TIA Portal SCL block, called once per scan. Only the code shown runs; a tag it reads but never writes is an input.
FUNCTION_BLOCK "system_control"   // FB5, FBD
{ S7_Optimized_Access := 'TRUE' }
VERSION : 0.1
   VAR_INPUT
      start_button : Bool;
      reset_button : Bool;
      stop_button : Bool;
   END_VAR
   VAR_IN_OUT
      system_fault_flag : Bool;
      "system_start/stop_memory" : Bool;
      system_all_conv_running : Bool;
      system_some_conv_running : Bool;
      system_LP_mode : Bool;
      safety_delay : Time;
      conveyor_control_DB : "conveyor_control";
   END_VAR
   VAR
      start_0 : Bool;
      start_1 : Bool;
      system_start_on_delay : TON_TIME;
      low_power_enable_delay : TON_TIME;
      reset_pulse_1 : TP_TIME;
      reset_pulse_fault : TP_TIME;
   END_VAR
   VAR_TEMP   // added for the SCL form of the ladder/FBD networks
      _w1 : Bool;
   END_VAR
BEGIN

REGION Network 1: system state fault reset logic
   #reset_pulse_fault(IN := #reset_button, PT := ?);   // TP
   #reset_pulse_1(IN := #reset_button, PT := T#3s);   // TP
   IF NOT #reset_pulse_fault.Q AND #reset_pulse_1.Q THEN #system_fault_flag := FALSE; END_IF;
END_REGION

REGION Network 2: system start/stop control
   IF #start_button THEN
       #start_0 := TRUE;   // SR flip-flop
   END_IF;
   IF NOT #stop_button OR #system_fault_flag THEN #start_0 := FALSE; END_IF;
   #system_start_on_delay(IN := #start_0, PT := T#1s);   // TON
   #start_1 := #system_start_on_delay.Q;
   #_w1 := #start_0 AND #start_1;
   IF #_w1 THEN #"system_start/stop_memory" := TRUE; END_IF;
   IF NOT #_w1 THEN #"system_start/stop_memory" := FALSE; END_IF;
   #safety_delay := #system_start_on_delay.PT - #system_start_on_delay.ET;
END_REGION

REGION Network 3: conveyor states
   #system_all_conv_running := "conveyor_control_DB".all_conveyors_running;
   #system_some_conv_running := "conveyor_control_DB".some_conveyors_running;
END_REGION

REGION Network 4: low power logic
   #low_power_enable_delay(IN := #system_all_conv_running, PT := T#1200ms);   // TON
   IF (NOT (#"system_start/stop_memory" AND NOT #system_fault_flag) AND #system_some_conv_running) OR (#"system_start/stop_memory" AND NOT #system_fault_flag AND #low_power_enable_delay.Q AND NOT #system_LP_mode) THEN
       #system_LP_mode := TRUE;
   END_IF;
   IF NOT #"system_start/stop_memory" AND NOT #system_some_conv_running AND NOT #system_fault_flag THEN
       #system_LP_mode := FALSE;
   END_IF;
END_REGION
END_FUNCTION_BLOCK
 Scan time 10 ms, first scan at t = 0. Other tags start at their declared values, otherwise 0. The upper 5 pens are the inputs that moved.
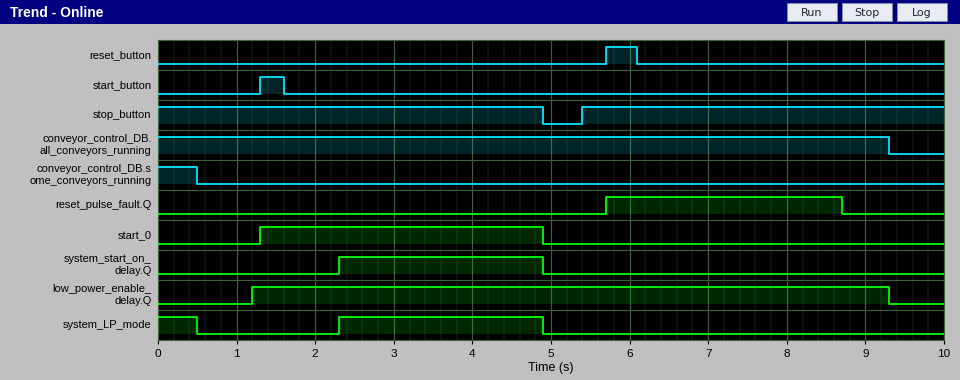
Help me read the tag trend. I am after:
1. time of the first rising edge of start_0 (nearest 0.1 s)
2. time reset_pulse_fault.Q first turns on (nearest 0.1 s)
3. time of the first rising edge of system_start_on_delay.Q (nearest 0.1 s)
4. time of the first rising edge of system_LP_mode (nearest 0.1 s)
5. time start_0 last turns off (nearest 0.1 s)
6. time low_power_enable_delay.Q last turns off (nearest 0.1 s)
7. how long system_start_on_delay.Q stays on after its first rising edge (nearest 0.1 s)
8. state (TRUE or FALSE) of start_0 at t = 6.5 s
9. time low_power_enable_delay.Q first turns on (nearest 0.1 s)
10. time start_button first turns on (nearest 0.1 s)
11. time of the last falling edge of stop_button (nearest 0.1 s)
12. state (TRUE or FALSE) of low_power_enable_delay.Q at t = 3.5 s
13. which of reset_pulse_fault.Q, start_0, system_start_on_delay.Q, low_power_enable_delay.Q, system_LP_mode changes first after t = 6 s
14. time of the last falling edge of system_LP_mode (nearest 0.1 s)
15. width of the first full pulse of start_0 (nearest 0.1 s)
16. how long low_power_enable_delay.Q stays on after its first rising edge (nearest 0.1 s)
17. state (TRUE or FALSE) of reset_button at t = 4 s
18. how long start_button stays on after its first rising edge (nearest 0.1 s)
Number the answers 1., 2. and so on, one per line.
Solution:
1. 1.3 s
2. 5.7 s
3. 2.3 s
4. 2.3 s
5. 4.9 s
6. 9.3 s
7. 2.6 s
8. FALSE
9. 1.2 s
10. 1.3 s
11. 4.9 s
12. TRUE
13. reset_pulse_fault.Q
14. 4.9 s
15. 3.6 s
16. 8.1 s
17. FALSE
18. 0.3 s
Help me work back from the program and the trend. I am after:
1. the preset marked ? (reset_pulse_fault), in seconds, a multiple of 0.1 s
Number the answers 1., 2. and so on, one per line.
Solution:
1. 3.0 s
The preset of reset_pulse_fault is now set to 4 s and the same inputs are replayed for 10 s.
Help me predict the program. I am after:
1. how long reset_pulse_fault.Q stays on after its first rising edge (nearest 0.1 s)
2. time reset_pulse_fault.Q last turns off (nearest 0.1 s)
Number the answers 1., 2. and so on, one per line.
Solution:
1. 4.0 s
2. 9.7 s
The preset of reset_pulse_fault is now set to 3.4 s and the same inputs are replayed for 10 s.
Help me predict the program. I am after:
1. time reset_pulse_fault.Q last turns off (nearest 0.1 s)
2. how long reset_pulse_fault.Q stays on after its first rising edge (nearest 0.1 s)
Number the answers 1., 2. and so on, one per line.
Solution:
1. 9.1 s
2. 3.4 s
